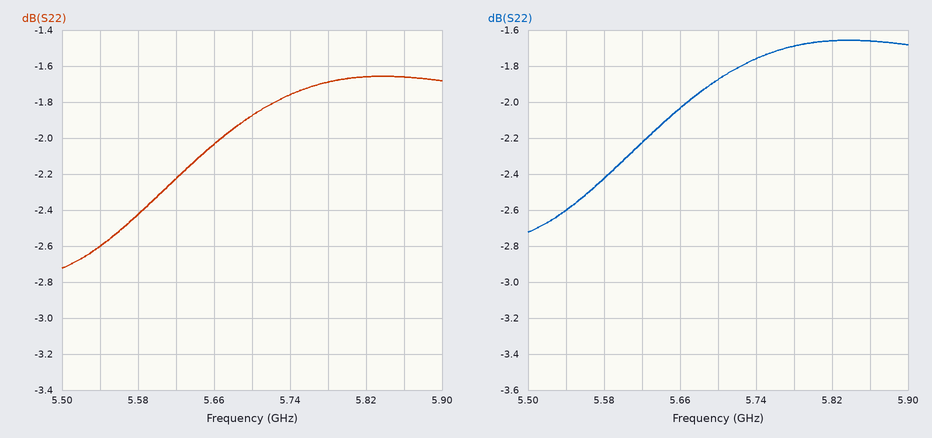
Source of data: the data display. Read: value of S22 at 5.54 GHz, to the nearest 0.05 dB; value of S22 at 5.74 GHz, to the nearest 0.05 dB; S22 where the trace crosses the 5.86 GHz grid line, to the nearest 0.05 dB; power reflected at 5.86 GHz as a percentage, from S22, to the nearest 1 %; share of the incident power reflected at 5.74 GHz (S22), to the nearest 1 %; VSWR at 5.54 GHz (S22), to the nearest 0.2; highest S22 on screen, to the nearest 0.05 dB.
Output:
-2.60 dB
-1.75 dB
-1.65 dB
68 %
67 %
6.8
-1.65 dB
